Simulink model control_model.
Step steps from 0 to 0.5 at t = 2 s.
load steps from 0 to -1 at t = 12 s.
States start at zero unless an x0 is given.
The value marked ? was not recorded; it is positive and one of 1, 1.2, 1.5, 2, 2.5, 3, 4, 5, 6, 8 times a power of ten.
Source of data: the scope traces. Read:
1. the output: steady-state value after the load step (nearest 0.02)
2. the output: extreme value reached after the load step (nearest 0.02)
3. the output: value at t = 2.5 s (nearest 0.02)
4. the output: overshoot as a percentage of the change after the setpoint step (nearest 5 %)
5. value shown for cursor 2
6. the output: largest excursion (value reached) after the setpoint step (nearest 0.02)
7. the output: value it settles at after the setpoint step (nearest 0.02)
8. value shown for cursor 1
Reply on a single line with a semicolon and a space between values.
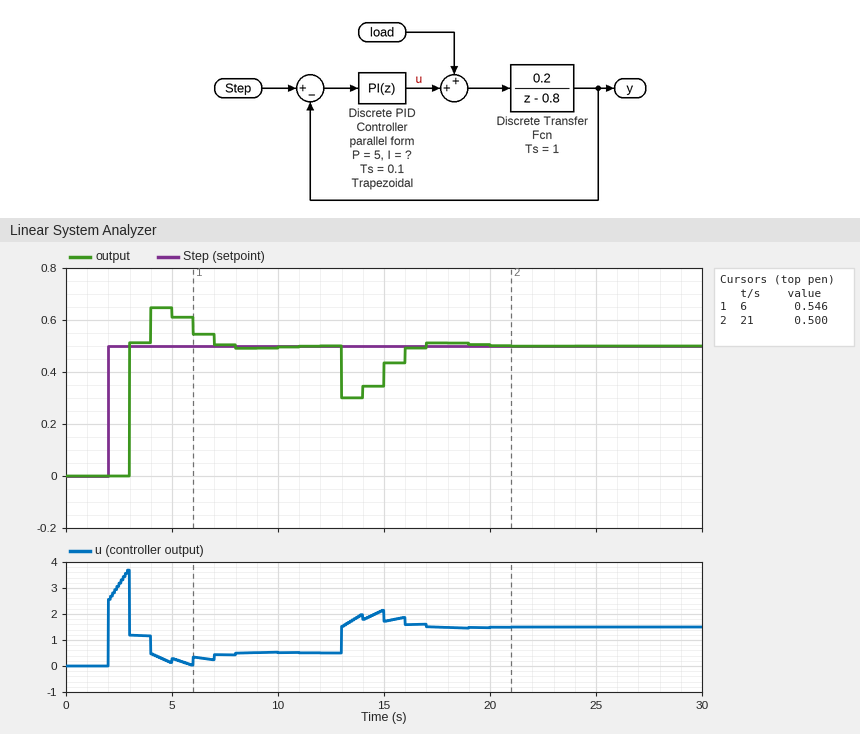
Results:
0.50; 0.30; 0.00; 30 %; 0.500; 0.64; 0.50; 0.546
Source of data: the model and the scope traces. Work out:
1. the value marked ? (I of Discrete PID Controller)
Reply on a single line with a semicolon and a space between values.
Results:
2.5
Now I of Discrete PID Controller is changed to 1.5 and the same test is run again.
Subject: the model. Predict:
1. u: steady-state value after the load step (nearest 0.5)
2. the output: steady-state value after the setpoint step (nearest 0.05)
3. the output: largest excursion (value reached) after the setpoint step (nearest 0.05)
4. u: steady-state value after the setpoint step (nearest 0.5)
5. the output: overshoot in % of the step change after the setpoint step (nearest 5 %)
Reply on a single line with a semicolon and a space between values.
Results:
1.5; 0.50; 0.55; 0.5; 10 %
